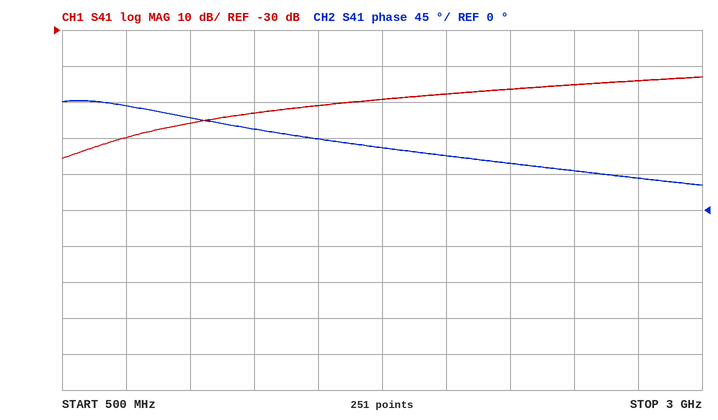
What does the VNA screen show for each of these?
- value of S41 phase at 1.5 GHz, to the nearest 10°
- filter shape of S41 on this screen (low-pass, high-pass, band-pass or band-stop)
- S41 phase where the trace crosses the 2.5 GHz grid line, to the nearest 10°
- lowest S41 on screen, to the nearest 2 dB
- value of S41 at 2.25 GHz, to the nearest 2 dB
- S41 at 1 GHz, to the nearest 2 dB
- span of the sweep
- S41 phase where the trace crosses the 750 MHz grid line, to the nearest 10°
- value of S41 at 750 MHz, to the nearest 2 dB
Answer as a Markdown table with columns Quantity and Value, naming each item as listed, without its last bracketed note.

| Quantity | Value |
|---|---|
| value of S41 phase at 1.5 GHz, to the nearest 10° | 90° |
| filter shape of S41 on this screen | high-pass |
| S41 phase where the trace crosses the 2.5 GHz grid line, to the nearest 10° | 50° |
| lowest S41 on screen, to the nearest 2 dB | -66 dB |
| value of S41 at 2.25 GHz, to the nearest 2 dB | -46 dB |
| S41 at 1 GHz, to the nearest 2 dB | -56 dB |
| span of the sweep | 2.5 GHz |
| S41 phase where the trace crosses the 750 MHz grid line, to the nearest 10° | 130° |
| value of S41 at 750 MHz, to the nearest 2 dB | -60 dB |
